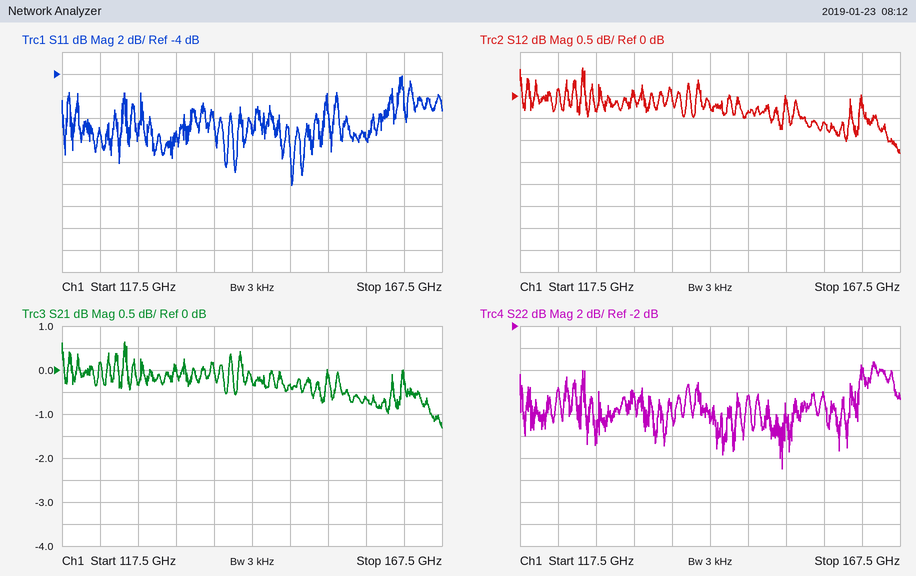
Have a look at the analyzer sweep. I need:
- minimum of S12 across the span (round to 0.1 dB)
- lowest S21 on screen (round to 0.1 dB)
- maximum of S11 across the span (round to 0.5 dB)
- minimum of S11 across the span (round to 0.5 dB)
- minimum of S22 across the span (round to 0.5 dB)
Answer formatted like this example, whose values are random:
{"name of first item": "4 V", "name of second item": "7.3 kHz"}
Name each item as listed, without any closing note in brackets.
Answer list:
{"minimum of S12 across the span": "-1.3 dB", "lowest S21 on screen": "-1.3 dB", "maximum of S11 across the span": "-4.0 dB", "minimum of S11 across the span": "-14.0 dB", "minimum of S22 across the span": "-15.0 dB"}
